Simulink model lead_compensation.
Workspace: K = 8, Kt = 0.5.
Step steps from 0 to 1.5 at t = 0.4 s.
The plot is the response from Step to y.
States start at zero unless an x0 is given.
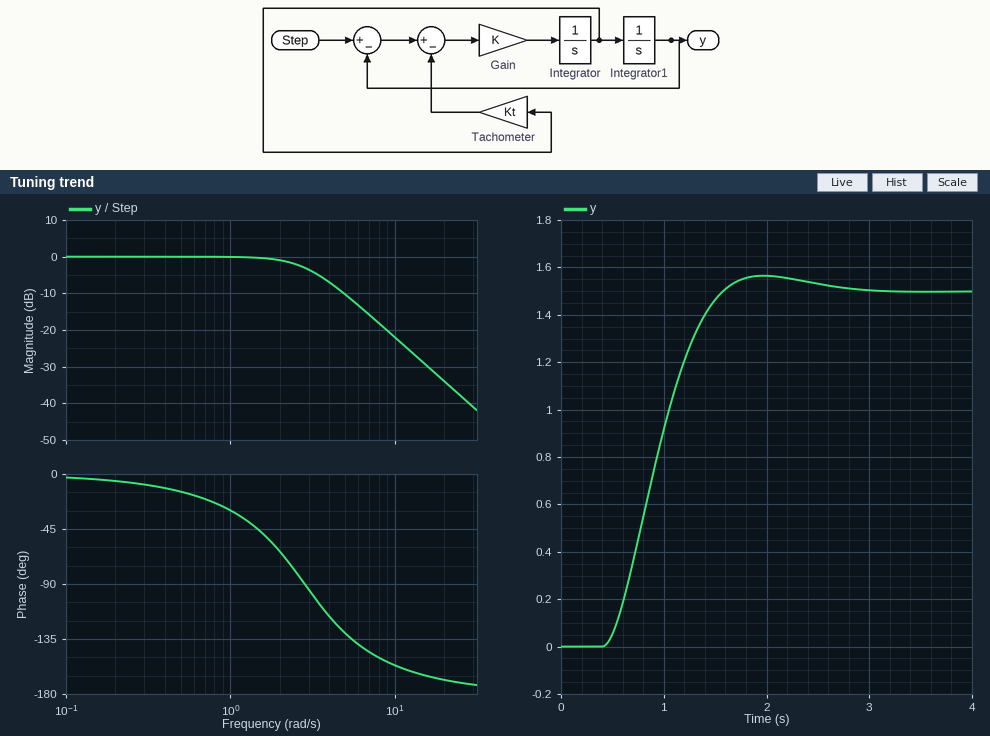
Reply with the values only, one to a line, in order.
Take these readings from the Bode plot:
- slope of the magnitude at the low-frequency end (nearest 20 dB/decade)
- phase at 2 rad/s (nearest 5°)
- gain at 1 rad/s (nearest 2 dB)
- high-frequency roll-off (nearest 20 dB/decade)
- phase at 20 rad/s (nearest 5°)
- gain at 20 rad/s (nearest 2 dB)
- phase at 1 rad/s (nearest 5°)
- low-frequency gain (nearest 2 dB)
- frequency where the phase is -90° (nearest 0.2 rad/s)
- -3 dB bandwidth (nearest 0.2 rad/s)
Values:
0 dB/decade
-65°
0 dB
-40 dB/decade
-170°
-34 dB
-30°
0 dB
2.8 rad/s
2.8 rad/s
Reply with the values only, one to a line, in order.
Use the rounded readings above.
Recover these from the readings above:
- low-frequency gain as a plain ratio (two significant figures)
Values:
1.0
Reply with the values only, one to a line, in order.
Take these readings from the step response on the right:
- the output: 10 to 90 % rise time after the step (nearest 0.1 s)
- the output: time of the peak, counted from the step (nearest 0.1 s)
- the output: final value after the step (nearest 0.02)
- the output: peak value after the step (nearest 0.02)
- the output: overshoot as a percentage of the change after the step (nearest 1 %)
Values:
0.8 s
1.6 s
1.50
1.56
4 %
